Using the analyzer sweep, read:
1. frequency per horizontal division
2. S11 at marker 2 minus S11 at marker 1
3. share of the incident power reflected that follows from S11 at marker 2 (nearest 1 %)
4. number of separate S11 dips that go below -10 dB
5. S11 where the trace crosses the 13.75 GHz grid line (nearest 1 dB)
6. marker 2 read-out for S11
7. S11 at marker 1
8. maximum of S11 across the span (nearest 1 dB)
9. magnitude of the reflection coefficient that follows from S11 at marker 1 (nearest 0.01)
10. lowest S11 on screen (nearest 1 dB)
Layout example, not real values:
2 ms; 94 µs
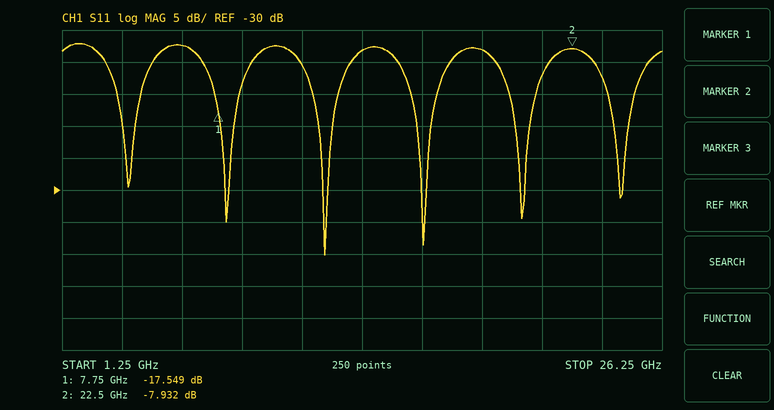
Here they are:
2.5 GHz; 9.617 dB; 16 %; 6; -8 dB; -7.932 dB; -17.549 dB; -7 dB; 0.13; -40 dB
